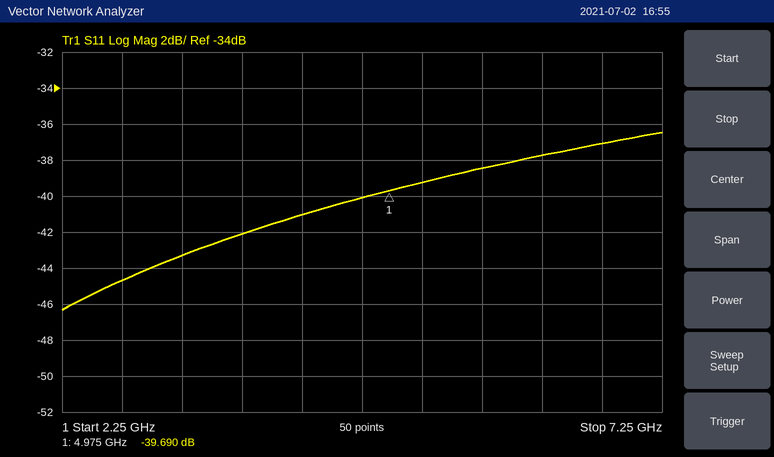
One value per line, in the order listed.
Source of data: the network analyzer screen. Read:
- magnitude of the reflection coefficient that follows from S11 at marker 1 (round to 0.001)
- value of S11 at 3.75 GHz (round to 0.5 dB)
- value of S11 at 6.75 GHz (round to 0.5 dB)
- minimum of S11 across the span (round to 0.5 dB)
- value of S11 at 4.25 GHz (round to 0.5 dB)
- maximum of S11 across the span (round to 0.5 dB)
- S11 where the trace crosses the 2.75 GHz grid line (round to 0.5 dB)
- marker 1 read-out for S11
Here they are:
0.010
-42.0 dB
-37.0 dB
-46.5 dB
-41.0 dB
-36.5 dB
-44.5 dB
-39.690 dB
